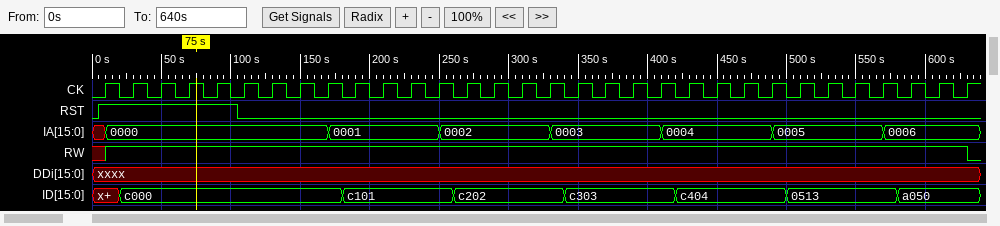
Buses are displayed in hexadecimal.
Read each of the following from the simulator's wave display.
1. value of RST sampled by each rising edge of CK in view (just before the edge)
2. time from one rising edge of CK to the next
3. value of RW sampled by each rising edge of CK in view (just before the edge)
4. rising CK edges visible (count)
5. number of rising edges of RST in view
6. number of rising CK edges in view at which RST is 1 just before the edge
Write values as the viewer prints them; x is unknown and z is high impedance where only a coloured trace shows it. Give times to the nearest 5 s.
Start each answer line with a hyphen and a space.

- 1 1 1 1 1 0 0 0 0 0 0 0 0 0 0 0 0 0 0 0 0 0 0 0 0 0 0 0 0 0 0 0
- 20 s
- x 1 1 1 1 1 1 1 1 1 1 1 1 1 1 1 1 1 1 1 1 1 1 1 1 1 1 1 1 1 1 1
- 32
- 1
- 5
